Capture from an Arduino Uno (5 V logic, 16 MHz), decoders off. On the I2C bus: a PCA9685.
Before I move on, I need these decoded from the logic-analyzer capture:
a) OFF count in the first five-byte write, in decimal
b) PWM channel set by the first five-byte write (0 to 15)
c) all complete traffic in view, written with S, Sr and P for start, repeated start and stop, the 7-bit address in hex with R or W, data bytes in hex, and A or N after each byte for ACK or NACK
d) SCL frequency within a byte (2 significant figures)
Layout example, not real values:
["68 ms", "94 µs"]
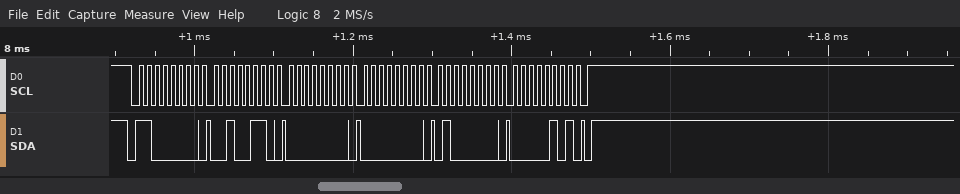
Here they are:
["1344", "8", "S 60W A 26 A 00 A 00 A 40 A 05 A P", "100 kHz"]
